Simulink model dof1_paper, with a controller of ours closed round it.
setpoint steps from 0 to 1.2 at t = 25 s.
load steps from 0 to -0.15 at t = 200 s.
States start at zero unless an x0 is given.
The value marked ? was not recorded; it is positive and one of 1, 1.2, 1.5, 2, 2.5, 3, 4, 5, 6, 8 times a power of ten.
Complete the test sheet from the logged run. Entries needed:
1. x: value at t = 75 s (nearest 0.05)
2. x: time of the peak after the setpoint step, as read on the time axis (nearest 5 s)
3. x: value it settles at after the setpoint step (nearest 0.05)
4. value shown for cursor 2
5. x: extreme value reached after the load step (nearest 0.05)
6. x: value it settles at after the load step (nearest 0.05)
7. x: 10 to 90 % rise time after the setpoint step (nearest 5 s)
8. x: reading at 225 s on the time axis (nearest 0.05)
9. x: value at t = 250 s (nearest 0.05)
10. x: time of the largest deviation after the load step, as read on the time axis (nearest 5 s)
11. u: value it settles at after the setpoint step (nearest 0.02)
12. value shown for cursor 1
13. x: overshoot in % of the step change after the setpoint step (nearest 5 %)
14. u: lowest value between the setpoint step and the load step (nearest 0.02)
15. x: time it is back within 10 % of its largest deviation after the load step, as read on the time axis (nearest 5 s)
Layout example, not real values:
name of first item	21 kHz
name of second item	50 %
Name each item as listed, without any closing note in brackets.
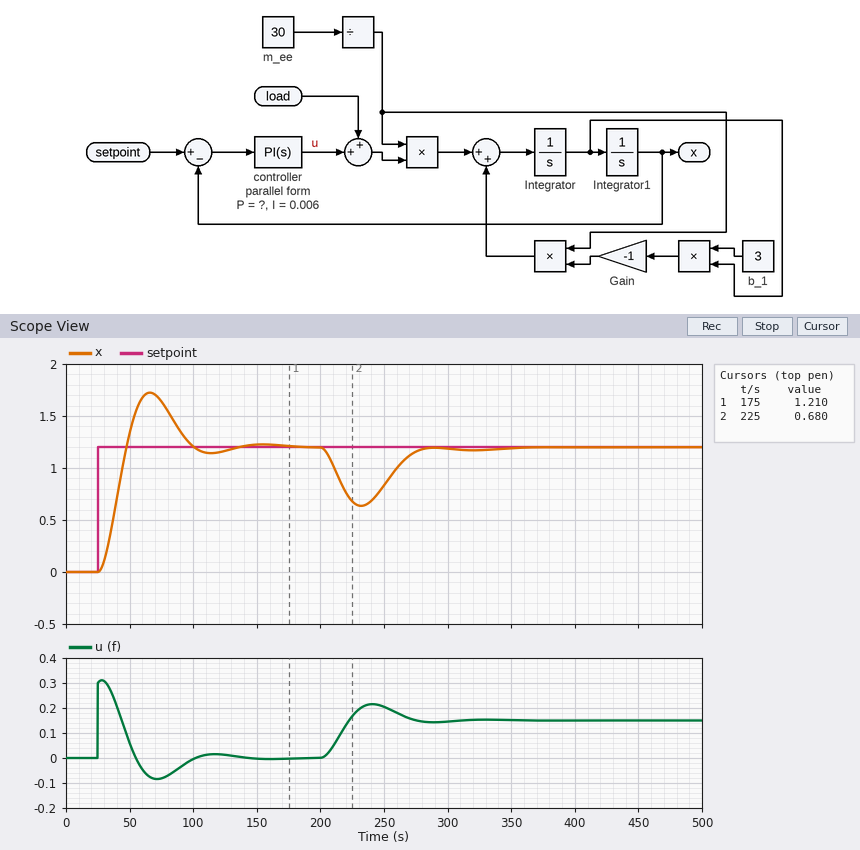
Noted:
x: value at t = 75 s	1.65
x: time of the peak after the setpoint step, as read on the time axis	65 s
x: value it settles at after the setpoint step	1.20
value shown for cursor 2	0.680
x: extreme value reached after the load step	0.65
x: value it settles at after the load step	1.20
x: 10 to 90 % rise time after the setpoint step	15 s
x: reading at 225 s on the time axis	0.70
x: value at t = 250 s	0.85
x: time of the largest deviation after the load step, as read on the time axis	230 s
u: value it settles at after the setpoint step	0.00
value shown for cursor 1	1.210
x: overshoot in % of the step change after the setpoint step	45 %
u: lowest value between the setpoint step and the load step	-0.08
x: time it is back within 10 % of its largest deviation after the load step, as read on the time axis	275 s
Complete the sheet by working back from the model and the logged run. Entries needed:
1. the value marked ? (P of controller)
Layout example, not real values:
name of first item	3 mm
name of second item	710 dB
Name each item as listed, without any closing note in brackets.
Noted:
the value marked ?	0.25
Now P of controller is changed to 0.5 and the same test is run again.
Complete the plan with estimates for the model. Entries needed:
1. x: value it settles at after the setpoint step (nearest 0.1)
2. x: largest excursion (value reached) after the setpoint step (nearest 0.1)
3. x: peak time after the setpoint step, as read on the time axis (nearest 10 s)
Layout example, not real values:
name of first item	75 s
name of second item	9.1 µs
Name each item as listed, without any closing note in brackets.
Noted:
x: value it settles at after the setpoint step	1.2
x: largest excursion (value reached) after the setpoint step	1.7
x: peak time after the setpoint step, as read on the time axis	50 s
